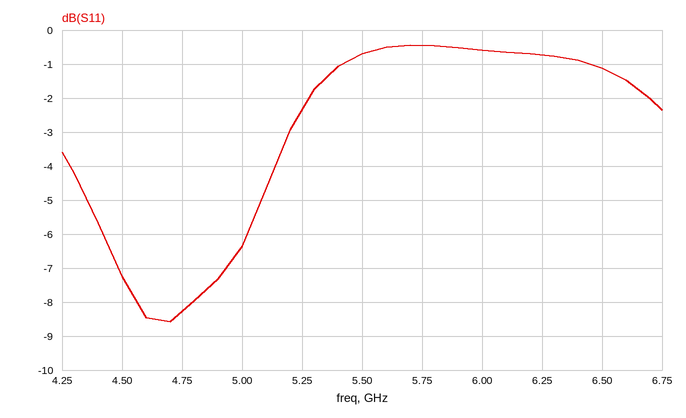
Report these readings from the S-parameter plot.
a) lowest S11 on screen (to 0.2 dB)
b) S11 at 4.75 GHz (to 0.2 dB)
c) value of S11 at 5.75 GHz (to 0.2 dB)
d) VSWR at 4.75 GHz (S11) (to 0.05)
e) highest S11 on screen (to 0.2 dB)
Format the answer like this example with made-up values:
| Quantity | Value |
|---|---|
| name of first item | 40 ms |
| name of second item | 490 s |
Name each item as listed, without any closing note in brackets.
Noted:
| Quantity | Value |
|---|---|
| lowest S11 on screen | -8.6 dB |
| S11 at 4.75 GHz | -8.2 dB |
| value of S11 at 5.75 GHz | -0.4 dB |
| VSWR at 4.75 GHz (S11) | 2.25 |
| highest S11 on screen | -0.4 dB |
